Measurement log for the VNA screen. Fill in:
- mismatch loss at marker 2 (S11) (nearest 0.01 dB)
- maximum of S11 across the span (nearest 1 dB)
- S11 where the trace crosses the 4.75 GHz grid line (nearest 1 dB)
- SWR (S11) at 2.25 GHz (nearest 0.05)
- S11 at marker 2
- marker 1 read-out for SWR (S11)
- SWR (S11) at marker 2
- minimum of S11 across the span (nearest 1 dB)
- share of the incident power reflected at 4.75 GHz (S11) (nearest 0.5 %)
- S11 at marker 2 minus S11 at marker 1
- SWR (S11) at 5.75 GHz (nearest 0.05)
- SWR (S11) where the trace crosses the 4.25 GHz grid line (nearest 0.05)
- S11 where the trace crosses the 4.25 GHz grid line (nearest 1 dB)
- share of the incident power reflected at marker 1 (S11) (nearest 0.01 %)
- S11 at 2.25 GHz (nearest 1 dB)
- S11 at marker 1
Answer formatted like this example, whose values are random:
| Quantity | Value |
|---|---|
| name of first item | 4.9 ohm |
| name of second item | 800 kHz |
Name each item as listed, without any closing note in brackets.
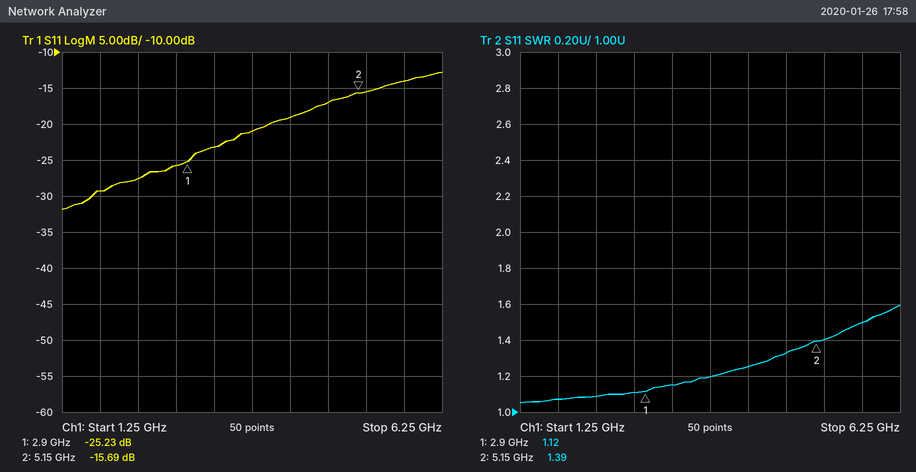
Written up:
| Quantity | Value |
|---|---|
| mismatch loss at marker 2 (S11) | 0.12 dB |
| maximum of S11 across the span | -13 dB |
| S11 where the trace crosses the 4.75 GHz grid line | -17 dB |
| SWR (S11) at 2.25 GHz | 1.10 |
| S11 at marker 2 | -15.69 dB |
| marker 1 read-out for SWR | 1.12 |
| SWR (S11) at marker 2 | 1.39 |
| minimum of S11 across the span | -32 dB |
| share of the incident power reflected at 4.75 GHz (S11) | 2.0 % |
| S11 at marker 2 minus S11 at marker 1 | 9.54 dB |
| SWR (S11) at 5.75 GHz | 1.50 |
| SWR (S11) where the trace crosses the 4.25 GHz grid line | 1.25 |
| S11 where the trace crosses the 4.25 GHz grid line | -19 dB |
| share of the incident power reflected at marker 1 (S11) | 0.30 % |
| S11 at 2.25 GHz | -28 dB |
| S11 at marker 1 | -25.23 dB |
